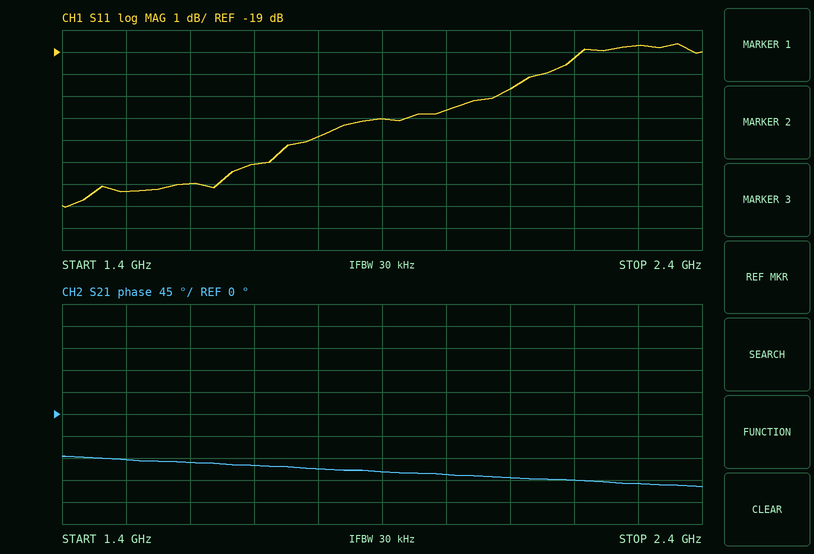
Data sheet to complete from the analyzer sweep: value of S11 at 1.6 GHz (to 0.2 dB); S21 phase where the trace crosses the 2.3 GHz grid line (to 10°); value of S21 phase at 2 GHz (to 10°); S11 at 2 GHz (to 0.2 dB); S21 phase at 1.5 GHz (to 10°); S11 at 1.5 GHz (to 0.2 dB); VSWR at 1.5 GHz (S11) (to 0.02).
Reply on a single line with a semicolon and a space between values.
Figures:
-25.0 dB; -140°; -120°; -21.6 dB; -90°; -25.4 dB; 1.12
